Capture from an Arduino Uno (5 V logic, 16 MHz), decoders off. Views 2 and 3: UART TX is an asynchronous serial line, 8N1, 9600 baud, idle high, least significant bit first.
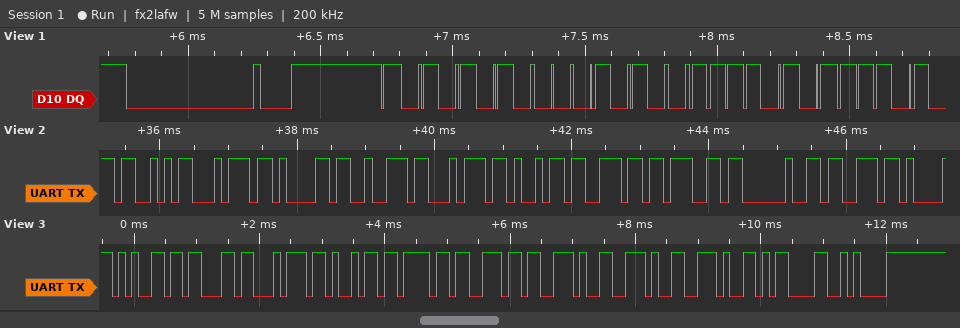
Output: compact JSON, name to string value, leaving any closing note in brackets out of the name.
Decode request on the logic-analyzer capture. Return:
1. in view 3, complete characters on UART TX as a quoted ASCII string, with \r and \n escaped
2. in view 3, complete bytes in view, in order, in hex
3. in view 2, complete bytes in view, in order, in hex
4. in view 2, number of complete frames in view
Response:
{"in view 3, complete characters on UART TX as a quoted ASCII string, with \\r and \\n escaped": "\"ection...\\r\\n\"", "in view 3, complete bytes in view, in order, in hex": "65 63 74 69 6F 6E 2E 2E 2E 0D 0A", "in view 2, complete bytes in view, in order, in hex": "53 74 61 72 74 69 6E 67 20 73", "in view 2, number of complete frames in view": "10"}
